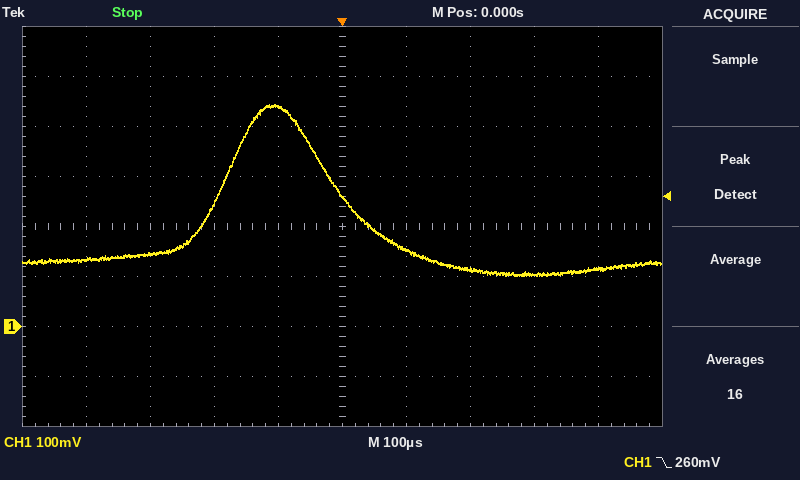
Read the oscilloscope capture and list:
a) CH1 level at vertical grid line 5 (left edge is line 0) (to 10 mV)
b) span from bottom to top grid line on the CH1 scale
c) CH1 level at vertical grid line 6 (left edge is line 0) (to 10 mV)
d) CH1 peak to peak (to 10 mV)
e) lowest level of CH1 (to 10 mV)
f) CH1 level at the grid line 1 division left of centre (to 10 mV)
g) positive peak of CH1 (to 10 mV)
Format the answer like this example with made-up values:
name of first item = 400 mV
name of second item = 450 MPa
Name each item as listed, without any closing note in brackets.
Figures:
CH1 level at vertical grid line 5 (left edge is line 0) = 260 mV
span from bottom to top grid line on the CH1 scale = 800 mV
CH1 level at vertical grid line 6 (left edge is line 0) = 150 mV
CH1 peak to peak = 340 mV
lowest level of CH1 = 100 mV
CH1 level at the grid line 1 division left of centre = 440 mV
positive peak of CH1 = 440 mV
